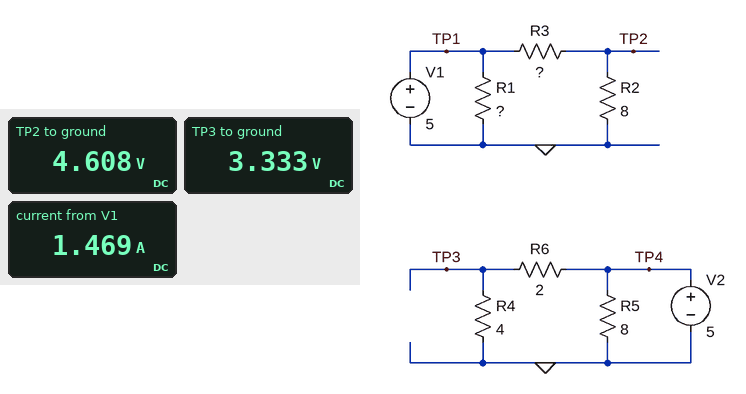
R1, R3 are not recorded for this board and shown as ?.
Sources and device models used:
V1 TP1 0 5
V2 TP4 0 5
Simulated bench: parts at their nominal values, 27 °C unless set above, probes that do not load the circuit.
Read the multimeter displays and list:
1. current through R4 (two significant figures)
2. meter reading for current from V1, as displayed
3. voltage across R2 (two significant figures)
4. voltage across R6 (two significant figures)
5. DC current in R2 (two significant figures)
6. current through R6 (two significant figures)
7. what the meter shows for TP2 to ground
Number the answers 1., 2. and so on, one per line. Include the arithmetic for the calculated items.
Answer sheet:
1. (3.333 V) / 4 Ω = 830 mA
2. 1.469 A
3. 4.608 V = 4.6 V
4. 5 V - 3.333 V = 1.7 V
5. (4.608 V) / 8 Ω = 580 mA
6. (5 V - 3.333 V) / 2 Ω = 830 mA
7. 4.608 V
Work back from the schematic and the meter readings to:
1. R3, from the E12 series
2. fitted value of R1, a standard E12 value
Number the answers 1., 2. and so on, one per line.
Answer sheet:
1. 0.68 Ω
2. 5.6 Ω
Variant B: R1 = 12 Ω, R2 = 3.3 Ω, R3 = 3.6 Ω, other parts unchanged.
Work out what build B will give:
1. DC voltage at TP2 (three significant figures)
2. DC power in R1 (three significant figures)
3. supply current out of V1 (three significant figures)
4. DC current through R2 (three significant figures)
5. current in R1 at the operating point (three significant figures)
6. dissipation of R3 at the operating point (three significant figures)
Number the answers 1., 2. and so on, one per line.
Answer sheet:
1. 2.39 V
2. 2.08 W
3. 1.14 A
4. 725 mA
5. 417 mA
6. 1.89 W
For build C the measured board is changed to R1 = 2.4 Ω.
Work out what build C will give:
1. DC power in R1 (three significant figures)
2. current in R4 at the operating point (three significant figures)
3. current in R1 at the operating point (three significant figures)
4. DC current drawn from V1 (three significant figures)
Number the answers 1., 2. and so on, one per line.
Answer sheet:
1. 10.4 W
2. 833 mA
3. 2.08 A
4. 2.66 A
